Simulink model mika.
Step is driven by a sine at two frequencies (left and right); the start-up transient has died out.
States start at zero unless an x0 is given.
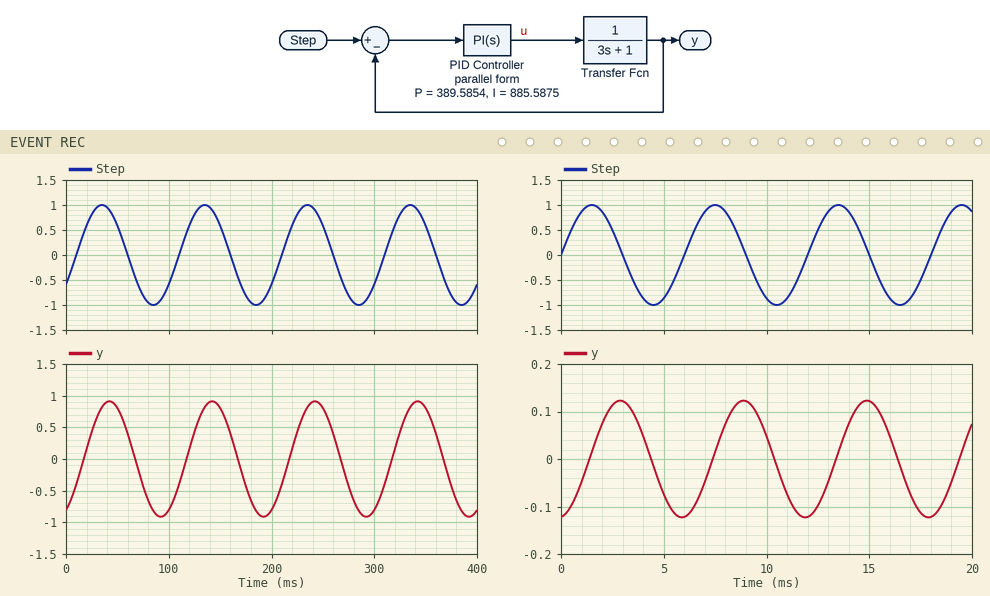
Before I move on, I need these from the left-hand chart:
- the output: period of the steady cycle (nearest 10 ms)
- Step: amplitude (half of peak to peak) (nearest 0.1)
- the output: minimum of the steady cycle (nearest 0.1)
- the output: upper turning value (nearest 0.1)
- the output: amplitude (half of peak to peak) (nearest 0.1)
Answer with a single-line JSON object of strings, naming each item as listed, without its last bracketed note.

{"the output: period of the steady cycle": "100 ms", "Step: amplitude (half of peak to peak)": "1.0", "the output: minimum of the steady cycle": "-0.9", "the output: upper turning value": "0.9", "the output: amplitude (half of peak to peak)": "0.9"}
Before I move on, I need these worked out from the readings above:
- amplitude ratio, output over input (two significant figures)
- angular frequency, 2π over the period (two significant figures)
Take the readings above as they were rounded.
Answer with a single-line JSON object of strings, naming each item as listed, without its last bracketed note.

{"amplitude ratio, output over input": "0.90", "angular frequency, 2π over the period": "0.063 rad/ms"}
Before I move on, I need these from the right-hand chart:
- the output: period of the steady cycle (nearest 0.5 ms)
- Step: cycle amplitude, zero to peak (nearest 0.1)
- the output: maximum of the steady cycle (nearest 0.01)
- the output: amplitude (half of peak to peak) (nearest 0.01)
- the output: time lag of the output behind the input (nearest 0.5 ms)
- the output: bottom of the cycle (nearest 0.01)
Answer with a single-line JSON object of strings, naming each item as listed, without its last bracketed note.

{"the output: period of the steady cycle": "6.0 ms", "Step: cycle amplitude, zero to peak": "1.0", "the output: maximum of the steady cycle": "0.12", "the output: amplitude (half of peak to peak)": "0.12", "the output: time lag of the output behind the input": "1.5 ms", "the output: bottom of the cycle": "-0.12"}
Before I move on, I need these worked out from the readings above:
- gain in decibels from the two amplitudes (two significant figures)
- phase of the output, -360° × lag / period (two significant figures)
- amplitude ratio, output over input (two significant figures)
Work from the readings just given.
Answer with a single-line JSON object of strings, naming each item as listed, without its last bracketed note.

{"gain in decibels from the two amplitudes": "-18 dB", "phase of the output, -360° × lag / period": "-90°", "amplitude ratio, output over input": "0.12"}
